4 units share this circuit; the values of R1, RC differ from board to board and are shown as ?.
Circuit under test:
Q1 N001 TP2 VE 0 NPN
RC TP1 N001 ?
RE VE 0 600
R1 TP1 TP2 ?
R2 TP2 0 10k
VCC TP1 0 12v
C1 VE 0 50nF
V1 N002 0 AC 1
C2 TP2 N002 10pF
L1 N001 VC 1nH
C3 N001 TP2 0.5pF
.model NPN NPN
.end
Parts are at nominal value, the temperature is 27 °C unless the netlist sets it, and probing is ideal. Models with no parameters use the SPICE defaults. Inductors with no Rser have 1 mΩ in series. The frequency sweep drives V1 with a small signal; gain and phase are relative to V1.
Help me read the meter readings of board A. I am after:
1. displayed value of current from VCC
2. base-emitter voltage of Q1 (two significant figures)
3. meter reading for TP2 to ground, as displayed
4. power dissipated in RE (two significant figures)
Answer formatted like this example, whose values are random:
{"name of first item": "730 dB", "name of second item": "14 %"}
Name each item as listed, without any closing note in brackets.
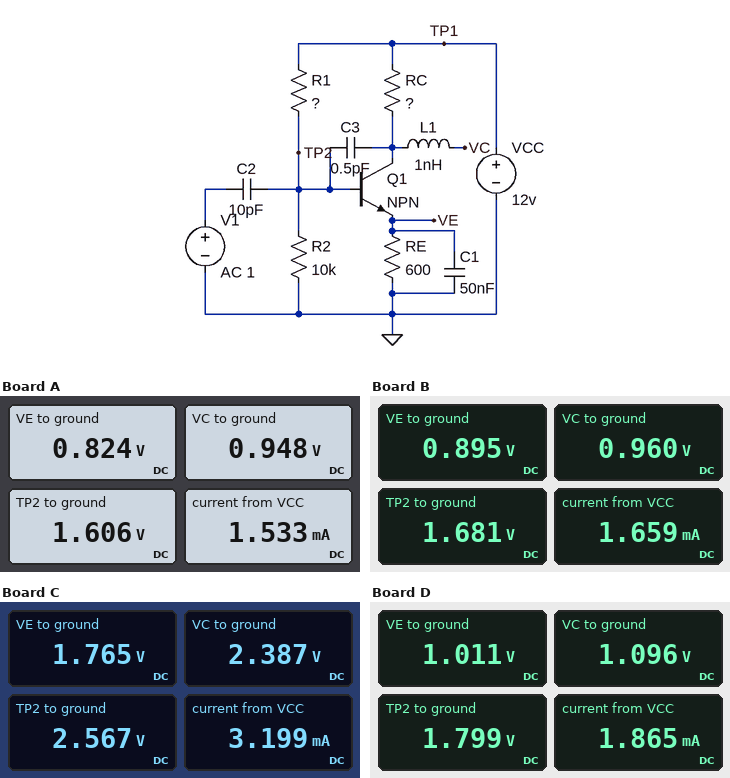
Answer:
{"displayed value of current from VCC": "1.533 mA", "base-emitter voltage of Q1": "780 mV", "meter reading for TP2 to ground, as displayed": "1.606 V", "power dissipated in RE": "1.1 mW"}
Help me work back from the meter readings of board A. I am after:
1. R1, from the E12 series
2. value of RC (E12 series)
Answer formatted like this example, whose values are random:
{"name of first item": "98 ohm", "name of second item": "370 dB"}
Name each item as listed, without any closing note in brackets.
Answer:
{"R1, from the E12 series": "56 kΩ", "value of RC": "8.2 kΩ"}
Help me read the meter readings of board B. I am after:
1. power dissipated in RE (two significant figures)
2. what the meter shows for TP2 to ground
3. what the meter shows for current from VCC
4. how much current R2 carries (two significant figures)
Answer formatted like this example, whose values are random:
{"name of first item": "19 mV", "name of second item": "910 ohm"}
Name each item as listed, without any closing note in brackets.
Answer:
{"power dissipated in RE": "1.3 mW", "what the meter shows for TP2 to ground": "1.681 V", "what the meter shows for current from VCC": "1.659 mA", "how much current R2 carries": "170 µA"}
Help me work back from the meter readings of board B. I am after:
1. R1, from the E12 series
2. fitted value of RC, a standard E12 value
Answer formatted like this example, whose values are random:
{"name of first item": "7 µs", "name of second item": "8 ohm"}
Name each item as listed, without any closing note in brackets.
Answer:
{"R1, from the E12 series": "33 kΩ", "fitted value of RC, a standard E12 value": "8.2 kΩ"}
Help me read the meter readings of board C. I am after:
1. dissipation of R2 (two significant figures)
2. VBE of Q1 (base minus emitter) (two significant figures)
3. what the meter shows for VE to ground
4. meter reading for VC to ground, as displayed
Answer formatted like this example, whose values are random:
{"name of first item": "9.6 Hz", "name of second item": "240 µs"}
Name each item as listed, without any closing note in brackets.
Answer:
{"dissipation of R2": "660 µW", "VBE of Q1 (base minus emitter)": "800 mV", "what the meter shows for VE to ground": "1.765 V", "meter reading for VC to ground, as displayed": "2.387 V"}
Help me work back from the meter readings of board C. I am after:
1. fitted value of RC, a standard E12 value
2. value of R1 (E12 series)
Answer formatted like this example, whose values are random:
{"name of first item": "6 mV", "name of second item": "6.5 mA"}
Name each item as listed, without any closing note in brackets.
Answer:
{"fitted value of RC, a standard E12 value": "3.3 kΩ", "value of R1": "33 kΩ"}
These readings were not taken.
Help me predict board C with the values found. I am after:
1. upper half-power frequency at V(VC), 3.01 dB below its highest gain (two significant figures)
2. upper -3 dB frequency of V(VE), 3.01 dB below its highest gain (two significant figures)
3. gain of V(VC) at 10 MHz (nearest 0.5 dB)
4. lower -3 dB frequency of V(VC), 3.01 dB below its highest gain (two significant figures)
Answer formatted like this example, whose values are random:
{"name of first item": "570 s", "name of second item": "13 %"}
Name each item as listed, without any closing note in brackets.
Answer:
{"upper half-power frequency at V(VC), 3.01 dB below its highest gain": "1.9 GHz", "upper -3 dB frequency of V(VE), 3.01 dB below its highest gain": "1.1 MHz", "gain of V(VC) at 10 MHz": "25.5 dB", "lower -3 dB frequency of V(VC), 3.01 dB below its highest gain": "990 kHz"}
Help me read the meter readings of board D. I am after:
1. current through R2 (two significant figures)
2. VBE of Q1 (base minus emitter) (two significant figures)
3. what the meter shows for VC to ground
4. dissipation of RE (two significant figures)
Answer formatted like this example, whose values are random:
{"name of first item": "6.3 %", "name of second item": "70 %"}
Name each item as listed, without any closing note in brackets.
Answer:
{"current through R2": "180 µA", "VBE of Q1 (base minus emitter)": "790 mV", "what the meter shows for VC to ground": "1.096 V", "dissipation of RE": "1.7 mW"}
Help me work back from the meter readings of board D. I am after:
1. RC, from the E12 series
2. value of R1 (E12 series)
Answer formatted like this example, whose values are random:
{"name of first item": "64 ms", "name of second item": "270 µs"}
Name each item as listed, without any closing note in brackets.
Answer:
{"RC, from the E12 series": "6.8 kΩ", "value of R1": "39 kΩ"}
